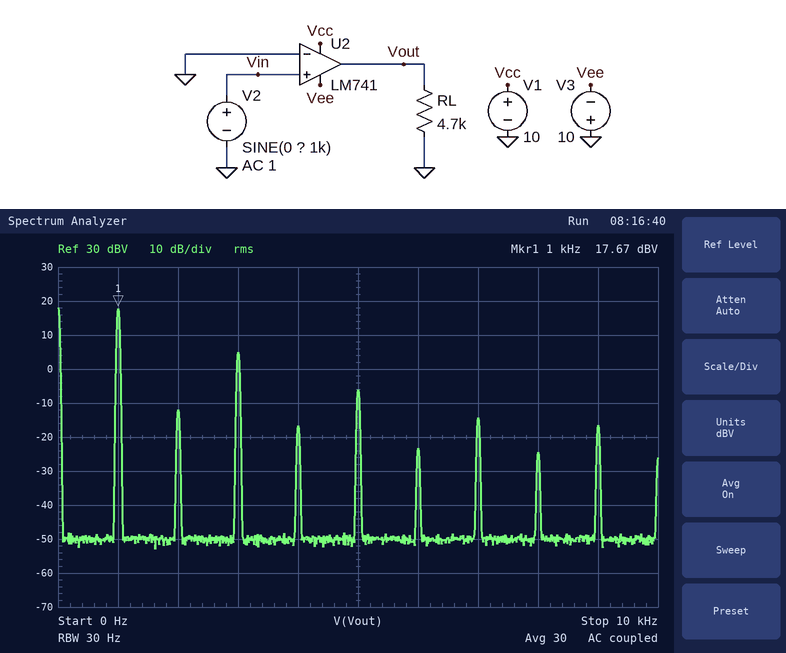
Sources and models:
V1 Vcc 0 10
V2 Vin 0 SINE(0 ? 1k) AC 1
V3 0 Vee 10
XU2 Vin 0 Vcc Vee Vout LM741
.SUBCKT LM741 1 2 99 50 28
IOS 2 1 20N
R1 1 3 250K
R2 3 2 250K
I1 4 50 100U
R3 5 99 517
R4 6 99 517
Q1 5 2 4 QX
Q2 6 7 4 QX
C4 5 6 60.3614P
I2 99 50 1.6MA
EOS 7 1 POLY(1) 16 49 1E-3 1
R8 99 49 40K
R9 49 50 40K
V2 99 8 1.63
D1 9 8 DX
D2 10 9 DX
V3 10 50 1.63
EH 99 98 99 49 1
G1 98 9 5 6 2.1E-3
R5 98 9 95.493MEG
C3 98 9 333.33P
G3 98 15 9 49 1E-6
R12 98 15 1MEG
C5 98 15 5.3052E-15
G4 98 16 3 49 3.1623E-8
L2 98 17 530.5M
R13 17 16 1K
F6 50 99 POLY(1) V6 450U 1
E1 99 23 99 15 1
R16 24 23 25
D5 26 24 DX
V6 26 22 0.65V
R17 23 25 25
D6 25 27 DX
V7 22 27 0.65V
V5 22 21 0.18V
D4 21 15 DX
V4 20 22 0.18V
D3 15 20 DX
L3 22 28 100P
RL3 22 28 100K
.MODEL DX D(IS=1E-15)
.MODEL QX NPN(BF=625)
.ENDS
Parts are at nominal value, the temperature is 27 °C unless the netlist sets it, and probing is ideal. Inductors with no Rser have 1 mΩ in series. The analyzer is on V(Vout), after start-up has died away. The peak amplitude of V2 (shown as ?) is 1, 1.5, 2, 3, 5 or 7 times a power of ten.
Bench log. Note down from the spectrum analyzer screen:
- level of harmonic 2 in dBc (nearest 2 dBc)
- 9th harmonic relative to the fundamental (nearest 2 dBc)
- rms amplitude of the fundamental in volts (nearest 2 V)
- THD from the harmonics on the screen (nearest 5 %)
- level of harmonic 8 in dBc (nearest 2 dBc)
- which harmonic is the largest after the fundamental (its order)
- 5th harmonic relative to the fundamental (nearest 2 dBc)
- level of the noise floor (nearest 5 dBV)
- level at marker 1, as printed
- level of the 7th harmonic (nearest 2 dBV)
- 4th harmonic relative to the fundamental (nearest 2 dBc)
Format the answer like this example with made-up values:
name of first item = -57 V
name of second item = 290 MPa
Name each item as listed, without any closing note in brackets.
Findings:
level of harmonic 2 in dBc = -30 dBc
9th harmonic relative to the fundamental = -34 dBc
rms amplitude of the fundamental in volts = 8 V
THD from the harmonics on the screen = 25 %
level of harmonic 8 in dBc = -42 dBc
which harmonic is the largest after the fundamental = 3
5th harmonic relative to the fundamental = -24 dBc
level of the noise floor = -50 dBV
level at marker 1, as printed = 17.67 dBV
level of the 7th harmonic = -14 dBV
4th harmonic relative to the fundamental = -34 dBc
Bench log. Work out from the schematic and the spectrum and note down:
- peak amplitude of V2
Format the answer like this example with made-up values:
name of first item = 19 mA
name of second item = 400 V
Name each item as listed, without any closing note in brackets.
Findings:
peak amplitude of V2 = 30 mV
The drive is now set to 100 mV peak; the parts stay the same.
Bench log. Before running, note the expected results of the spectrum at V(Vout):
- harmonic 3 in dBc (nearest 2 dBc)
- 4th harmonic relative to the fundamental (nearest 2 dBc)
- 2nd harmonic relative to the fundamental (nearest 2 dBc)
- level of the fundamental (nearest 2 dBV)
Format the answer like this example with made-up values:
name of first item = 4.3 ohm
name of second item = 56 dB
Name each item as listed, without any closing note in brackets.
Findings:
harmonic 3 in dBc = -10 dBc
4th harmonic relative to the fundamental = -42 dBc
2nd harmonic relative to the fundamental = -40 dBc
level of the fundamental = 18 dBV
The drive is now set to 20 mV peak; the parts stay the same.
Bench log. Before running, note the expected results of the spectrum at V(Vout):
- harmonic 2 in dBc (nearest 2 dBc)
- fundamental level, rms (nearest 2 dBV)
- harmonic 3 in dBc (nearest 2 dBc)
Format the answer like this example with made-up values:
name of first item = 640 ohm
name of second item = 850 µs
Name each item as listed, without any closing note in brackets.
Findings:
harmonic 2 in dBc = -26 dBc
fundamental level, rms = 18 dBV
harmonic 3 in dBc = -14 dBc
